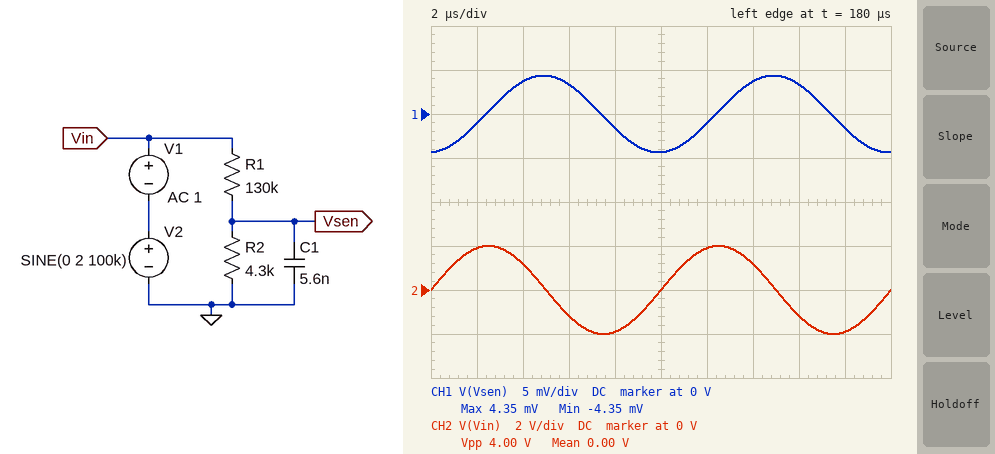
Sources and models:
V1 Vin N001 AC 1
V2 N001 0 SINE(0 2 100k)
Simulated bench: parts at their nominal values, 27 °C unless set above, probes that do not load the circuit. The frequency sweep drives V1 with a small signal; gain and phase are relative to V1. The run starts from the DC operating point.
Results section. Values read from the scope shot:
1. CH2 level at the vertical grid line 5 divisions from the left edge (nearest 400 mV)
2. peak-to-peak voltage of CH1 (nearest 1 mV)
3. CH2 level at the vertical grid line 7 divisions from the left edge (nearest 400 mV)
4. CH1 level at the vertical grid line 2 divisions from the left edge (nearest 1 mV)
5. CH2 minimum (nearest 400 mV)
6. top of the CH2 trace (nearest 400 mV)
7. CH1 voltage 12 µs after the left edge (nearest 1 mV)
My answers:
0 V
9 mV
1.2 V
4 mV
-2.0 V
2.0 V
-1 mV
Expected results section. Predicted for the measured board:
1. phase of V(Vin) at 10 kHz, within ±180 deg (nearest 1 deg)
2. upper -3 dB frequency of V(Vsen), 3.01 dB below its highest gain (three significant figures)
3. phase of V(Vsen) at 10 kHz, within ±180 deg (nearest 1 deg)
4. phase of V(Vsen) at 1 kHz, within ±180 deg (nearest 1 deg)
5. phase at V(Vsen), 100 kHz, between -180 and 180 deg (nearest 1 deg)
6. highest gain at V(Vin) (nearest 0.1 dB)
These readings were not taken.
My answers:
0 deg
6.83 kHz
-56 deg
-8 deg
-86 deg
0 dB
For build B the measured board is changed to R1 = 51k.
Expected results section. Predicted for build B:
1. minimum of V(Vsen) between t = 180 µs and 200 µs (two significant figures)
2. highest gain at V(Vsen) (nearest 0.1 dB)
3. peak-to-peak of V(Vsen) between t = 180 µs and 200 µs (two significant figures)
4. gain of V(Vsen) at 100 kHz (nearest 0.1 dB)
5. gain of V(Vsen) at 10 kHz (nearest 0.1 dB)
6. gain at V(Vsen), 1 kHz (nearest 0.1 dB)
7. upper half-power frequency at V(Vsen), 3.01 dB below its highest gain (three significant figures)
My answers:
-11 mV
-22.2 dB
22 mV
-45.1 dB
-26.9 dB
-22.3 dB
7.17 kHz
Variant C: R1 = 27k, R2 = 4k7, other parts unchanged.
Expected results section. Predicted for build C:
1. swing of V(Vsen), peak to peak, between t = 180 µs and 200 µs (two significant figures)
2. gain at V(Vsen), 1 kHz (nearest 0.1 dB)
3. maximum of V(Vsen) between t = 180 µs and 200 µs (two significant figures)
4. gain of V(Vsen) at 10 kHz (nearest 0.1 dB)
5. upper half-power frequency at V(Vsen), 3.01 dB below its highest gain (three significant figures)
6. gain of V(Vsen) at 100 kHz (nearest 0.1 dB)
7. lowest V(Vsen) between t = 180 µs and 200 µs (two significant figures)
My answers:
42 mV
-16.7 dB
21 mV
-21.3 dB
7.10 kHz
-39.6 dB
-21 mV
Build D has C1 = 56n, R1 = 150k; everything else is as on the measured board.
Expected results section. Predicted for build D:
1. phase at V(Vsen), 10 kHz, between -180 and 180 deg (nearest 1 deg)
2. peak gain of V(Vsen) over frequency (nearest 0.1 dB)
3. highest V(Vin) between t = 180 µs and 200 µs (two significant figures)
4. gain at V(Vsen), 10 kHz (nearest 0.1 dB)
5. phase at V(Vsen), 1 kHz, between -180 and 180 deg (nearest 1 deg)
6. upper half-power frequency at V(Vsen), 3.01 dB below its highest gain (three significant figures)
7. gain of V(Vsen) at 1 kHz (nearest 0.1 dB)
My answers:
-86 deg
-31.1 dB
2.0 V
-54.5 dB
-56 deg
680 Hz
-36.1 dB
